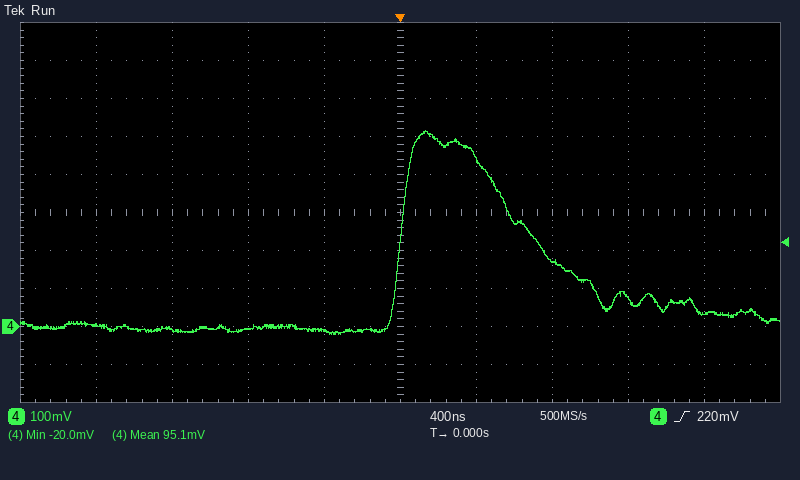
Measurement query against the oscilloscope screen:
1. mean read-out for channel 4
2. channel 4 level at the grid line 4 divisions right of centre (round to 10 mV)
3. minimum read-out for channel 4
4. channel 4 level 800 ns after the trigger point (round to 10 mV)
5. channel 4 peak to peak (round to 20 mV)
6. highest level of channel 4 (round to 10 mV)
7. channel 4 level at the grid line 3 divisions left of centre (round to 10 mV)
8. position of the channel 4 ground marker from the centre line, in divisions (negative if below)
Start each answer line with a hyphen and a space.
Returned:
- 95.1 mV
- 30 mV
- -20.0 mV
- 170 mV
- 540 mV
- 520 mV
- -10 mV
- -3.0 div
